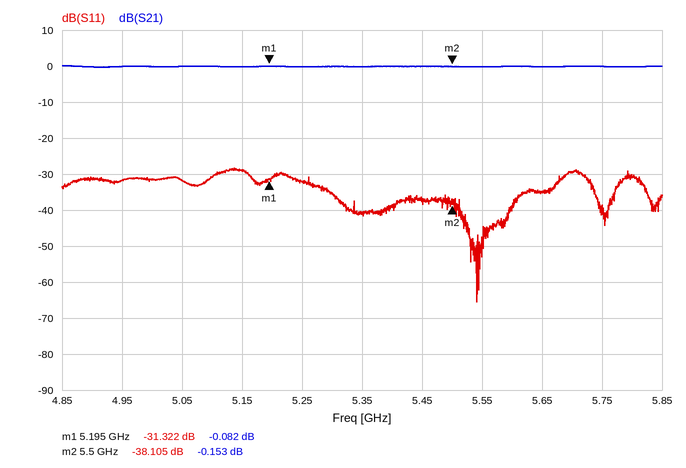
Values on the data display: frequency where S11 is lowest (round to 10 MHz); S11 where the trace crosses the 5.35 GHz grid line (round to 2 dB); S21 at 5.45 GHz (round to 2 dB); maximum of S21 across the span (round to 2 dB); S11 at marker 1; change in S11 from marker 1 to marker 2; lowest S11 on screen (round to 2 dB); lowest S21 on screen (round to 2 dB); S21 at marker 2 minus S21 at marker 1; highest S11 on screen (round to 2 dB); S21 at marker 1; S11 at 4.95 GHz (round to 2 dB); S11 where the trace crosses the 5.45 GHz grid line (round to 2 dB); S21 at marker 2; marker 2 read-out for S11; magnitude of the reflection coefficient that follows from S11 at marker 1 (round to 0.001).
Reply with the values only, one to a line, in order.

5.54 GHz
-40 dB
0 dB
0 dB
-31.322 dB
-6.783 dB
-66 dB
0 dB
-0.071 dB
-28 dB
-0.082 dB
-32 dB
-38 dB
-0.153 dB
-38.105 dB
0.027
